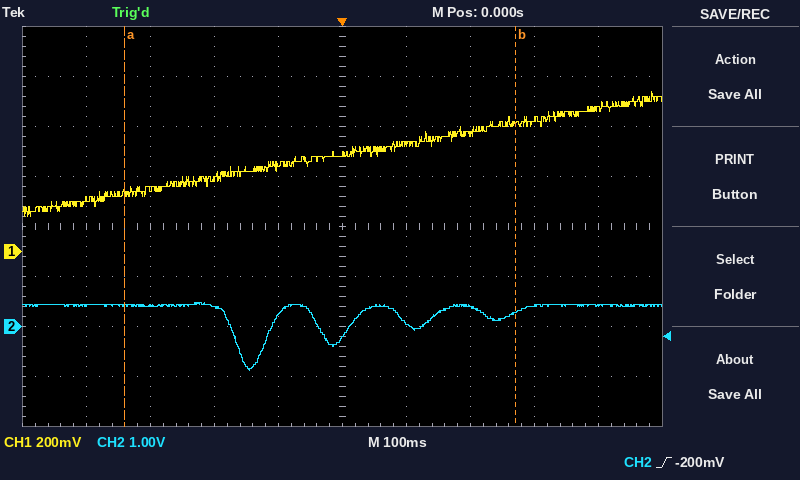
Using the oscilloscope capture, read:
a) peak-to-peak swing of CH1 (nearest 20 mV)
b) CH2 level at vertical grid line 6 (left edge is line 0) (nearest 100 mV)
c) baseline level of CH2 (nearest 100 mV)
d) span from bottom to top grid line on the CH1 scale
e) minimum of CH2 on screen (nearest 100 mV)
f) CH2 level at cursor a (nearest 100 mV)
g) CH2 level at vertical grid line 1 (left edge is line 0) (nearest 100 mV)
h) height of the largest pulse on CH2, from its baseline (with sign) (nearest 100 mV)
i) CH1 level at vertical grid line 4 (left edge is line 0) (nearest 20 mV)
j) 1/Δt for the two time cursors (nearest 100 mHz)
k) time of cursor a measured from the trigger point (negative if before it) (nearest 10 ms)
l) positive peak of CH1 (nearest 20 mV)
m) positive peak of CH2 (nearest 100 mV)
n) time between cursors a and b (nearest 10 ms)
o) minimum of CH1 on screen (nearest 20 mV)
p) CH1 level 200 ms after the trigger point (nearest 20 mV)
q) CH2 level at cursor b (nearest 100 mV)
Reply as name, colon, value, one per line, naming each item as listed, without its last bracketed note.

peak-to-peak swing of CH1: 500 mV
CH2 level at vertical grid line 6 (left edge is line 0): 100 mV
baseline level of CH2: 400 mV
span from bottom to top grid line on the CH1 scale: 1.6 V
minimum of CH2 on screen: -900 mV
CH2 level at cursor a: 400 mV
CH2 level at vertical grid line 1 (left edge is line 0): 400 mV
height of the largest pulse on CH2, from its baseline (with sign): -1.3 V
CH1 level at vertical grid line 4 (left edge is line 0): 340 mV
1/Δt for the two time cursors: 1.6 Hz
time of cursor a measured from the trigger point (negative if before it): -340 ms
positive peak of CH1: 640 mV
positive peak of CH2: 500 mV
time between cursors a and b: 610 ms
minimum of CH1 on screen: 140 mV
CH1 level 200 ms after the trigger point: 480 mV
CH2 level at cursor b: 300 mV
